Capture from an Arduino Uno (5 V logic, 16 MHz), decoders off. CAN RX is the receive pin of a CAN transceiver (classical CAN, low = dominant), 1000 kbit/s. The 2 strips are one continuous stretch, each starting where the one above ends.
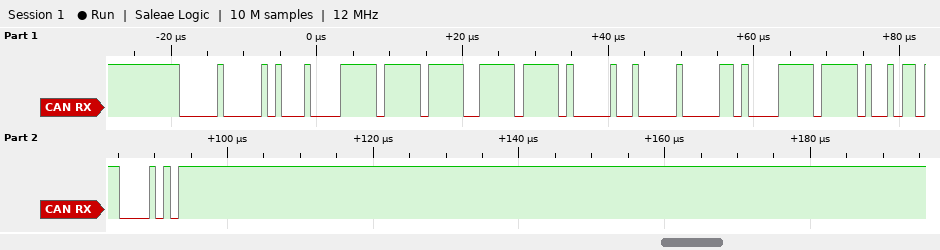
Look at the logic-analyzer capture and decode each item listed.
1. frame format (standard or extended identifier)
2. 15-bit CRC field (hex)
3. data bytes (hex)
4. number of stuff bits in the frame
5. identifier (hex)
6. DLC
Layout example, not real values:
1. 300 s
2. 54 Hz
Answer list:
1. standard
2. 0x16C2
3. 7F FF 7F F0 10 02 87 FF
4. 12
5. 0x001
6. 8
